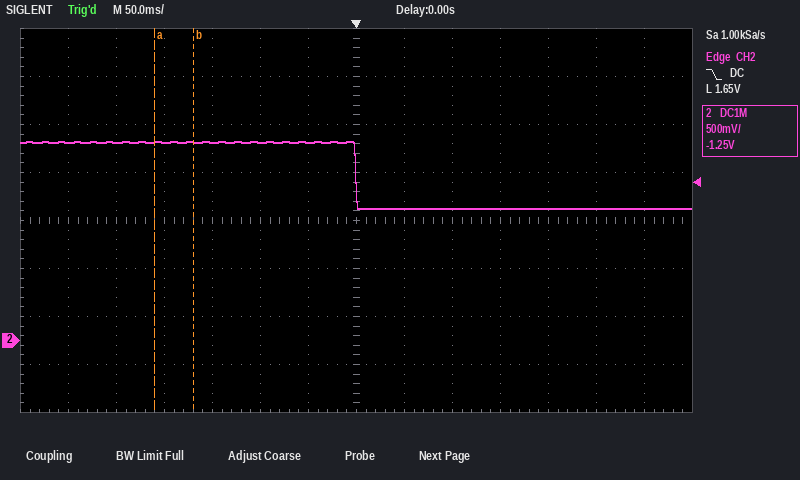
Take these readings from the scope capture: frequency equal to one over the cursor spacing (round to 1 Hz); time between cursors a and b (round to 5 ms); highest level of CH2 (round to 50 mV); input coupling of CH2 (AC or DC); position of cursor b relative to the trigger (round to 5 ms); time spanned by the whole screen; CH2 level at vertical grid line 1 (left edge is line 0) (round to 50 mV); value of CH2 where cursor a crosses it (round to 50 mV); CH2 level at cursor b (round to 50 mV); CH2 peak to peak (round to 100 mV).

25 Hz
40 ms
2.05 V
DC
-170 ms
700 ms
2.05 V
2.05 V
2.05 V
700 mV
